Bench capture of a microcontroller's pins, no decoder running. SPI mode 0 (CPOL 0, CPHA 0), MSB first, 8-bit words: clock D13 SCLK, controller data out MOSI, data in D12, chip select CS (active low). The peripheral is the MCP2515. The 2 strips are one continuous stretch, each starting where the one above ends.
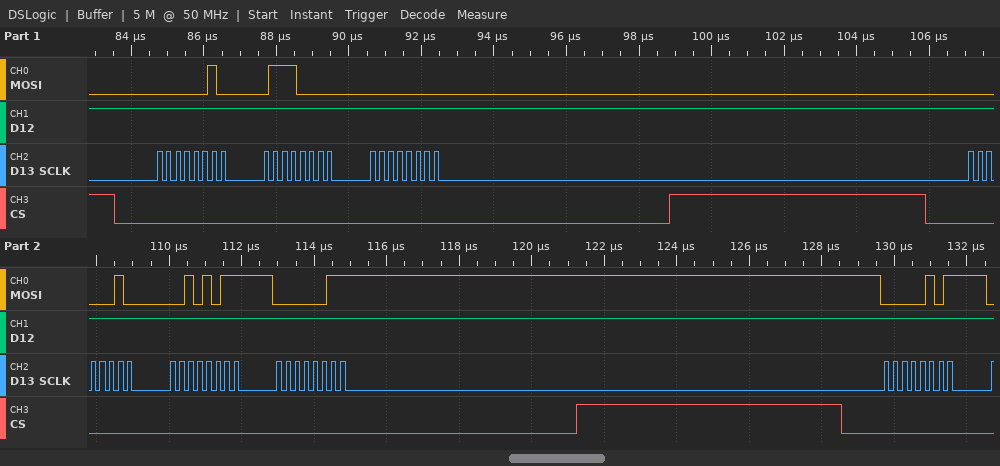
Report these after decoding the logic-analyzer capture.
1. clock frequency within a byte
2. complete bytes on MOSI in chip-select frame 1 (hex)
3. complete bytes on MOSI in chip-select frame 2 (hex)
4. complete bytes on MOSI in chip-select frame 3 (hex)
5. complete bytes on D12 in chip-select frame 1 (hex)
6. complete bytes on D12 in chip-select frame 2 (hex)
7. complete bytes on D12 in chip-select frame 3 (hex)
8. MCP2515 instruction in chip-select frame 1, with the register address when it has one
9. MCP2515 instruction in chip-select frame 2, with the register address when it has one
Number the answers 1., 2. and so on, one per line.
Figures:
1. 4 MHz
2. 02 70 00
3. 02 2B 03
4. 05
5. FF FF FF
6. FF FF FF
7. FF
8. WRITE 0x70
9. WRITE 0x2B
